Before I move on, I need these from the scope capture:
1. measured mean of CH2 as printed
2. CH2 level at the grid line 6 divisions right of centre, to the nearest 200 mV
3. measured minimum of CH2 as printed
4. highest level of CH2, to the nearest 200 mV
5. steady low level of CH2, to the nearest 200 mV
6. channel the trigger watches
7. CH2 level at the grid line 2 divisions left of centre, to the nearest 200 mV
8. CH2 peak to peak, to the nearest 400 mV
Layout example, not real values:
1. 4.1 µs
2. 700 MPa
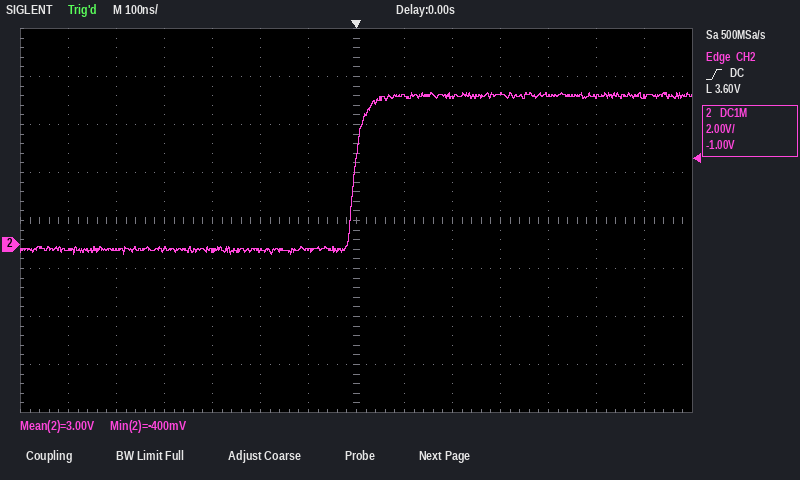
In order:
1. 3.00 V
2. 6.2 V
3. -400 mV
4. 6.4 V
5. -200 mV
6. CH2
7. -200 mV
8. 6.8 V
